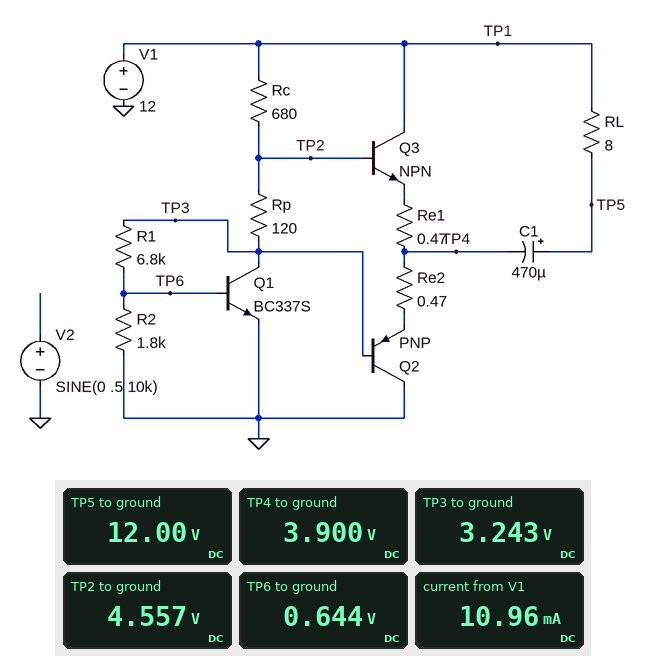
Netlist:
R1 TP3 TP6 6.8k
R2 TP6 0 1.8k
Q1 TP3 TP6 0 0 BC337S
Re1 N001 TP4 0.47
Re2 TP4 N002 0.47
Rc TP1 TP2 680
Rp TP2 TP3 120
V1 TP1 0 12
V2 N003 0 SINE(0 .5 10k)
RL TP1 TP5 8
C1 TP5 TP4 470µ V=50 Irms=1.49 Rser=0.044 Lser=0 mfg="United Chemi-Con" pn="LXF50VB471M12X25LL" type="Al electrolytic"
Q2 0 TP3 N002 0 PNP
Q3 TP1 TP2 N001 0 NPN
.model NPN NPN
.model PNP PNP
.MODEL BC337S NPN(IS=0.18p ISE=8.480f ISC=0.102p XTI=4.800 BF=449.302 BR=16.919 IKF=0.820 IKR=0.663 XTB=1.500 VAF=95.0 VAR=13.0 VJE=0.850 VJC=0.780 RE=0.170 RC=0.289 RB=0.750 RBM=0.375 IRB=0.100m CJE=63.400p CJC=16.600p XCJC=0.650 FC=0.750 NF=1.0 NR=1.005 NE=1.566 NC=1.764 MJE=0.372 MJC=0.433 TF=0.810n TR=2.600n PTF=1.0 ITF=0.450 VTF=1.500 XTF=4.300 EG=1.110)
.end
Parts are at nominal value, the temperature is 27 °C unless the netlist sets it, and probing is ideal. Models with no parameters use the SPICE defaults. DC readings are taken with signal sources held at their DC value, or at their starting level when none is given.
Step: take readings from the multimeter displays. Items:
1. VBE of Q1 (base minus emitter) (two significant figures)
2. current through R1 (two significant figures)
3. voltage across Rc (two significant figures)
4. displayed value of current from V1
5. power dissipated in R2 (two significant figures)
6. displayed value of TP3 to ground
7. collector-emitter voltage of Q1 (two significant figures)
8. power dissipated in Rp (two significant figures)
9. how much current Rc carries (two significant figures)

640 mV
380 µA
7.4 V
10.96 mA
230 µW
3.243 V
3.2 V
14 mW
11 mA
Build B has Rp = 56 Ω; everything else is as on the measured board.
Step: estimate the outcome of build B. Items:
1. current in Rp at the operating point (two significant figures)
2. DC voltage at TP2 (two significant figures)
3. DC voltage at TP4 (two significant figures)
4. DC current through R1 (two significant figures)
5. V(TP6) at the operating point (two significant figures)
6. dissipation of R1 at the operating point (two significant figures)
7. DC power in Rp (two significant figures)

12 mA
3.9 V
3.6 V
390 µA
650 mV
1.0 mW
7.9 mW
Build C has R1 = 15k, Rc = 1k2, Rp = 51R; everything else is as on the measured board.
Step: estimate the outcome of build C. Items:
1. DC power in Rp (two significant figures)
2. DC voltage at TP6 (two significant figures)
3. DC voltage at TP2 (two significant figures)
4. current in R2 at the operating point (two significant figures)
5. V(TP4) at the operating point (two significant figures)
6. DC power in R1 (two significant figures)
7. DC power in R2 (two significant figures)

1.2 mW
620 mV
6.2 V
340 µA
6.1 V
1.9 mW
210 µW
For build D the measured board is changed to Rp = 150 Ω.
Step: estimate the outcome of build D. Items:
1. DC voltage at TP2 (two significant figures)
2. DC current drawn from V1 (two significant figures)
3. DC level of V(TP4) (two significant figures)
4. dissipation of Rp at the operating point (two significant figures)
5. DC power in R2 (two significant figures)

4.8 V
12 mA
4.0 V
17 mW
230 µW
